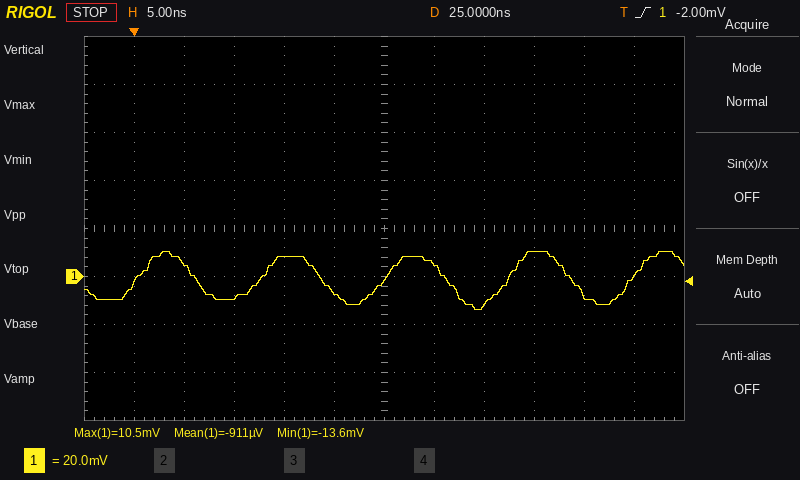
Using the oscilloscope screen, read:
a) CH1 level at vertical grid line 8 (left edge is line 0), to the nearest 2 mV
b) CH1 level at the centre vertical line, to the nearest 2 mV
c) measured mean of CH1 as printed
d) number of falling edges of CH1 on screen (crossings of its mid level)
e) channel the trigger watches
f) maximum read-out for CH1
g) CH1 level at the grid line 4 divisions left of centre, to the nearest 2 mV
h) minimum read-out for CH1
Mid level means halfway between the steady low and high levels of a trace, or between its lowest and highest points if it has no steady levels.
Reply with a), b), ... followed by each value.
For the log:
a) -12 mV
b) -2 mV
c) -911 µV
d) 4
e) CH1
f) 10.5 mV
g) 6 mV
h) -13.6 mV
